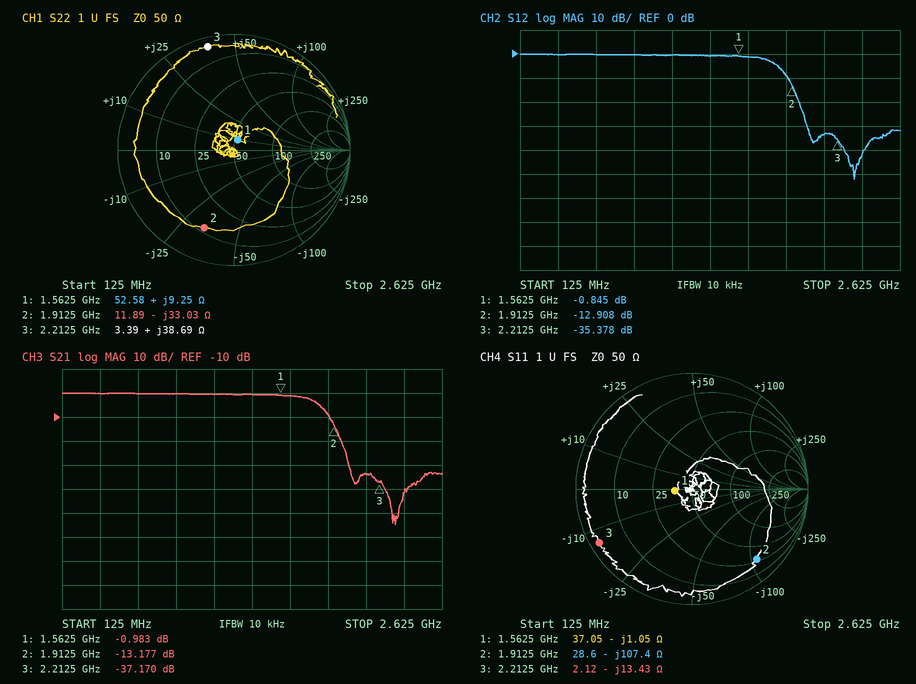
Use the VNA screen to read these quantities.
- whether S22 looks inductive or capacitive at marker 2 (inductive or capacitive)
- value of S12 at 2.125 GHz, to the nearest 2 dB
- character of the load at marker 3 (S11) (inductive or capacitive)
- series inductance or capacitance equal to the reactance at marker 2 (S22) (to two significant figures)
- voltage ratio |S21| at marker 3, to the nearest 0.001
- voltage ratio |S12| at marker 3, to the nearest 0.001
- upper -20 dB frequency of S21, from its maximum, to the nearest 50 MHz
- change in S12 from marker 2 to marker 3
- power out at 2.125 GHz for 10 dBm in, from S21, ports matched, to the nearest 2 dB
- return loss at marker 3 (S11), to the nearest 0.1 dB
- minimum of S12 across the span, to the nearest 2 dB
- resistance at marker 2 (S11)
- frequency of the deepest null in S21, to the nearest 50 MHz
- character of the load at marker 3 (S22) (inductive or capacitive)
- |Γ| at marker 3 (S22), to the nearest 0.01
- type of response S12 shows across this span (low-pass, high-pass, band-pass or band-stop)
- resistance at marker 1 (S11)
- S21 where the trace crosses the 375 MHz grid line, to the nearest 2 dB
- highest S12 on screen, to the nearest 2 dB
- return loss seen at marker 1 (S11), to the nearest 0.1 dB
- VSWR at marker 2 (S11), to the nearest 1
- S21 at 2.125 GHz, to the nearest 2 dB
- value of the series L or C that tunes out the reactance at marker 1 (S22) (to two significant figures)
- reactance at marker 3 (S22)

capacitive
-34 dB
capacitive
2.5 pF
0.014
0.017
1.95 GHz
-22.470 dB
-24 dBm
0.7 dB
-52 dB
28.6 Ω
2.30 GHz
inductive
0.92
low-pass
37.05 Ω
0 dB
0 dB
16.5 dB
10
-34 dB
11 pF
+38.69 Ω
